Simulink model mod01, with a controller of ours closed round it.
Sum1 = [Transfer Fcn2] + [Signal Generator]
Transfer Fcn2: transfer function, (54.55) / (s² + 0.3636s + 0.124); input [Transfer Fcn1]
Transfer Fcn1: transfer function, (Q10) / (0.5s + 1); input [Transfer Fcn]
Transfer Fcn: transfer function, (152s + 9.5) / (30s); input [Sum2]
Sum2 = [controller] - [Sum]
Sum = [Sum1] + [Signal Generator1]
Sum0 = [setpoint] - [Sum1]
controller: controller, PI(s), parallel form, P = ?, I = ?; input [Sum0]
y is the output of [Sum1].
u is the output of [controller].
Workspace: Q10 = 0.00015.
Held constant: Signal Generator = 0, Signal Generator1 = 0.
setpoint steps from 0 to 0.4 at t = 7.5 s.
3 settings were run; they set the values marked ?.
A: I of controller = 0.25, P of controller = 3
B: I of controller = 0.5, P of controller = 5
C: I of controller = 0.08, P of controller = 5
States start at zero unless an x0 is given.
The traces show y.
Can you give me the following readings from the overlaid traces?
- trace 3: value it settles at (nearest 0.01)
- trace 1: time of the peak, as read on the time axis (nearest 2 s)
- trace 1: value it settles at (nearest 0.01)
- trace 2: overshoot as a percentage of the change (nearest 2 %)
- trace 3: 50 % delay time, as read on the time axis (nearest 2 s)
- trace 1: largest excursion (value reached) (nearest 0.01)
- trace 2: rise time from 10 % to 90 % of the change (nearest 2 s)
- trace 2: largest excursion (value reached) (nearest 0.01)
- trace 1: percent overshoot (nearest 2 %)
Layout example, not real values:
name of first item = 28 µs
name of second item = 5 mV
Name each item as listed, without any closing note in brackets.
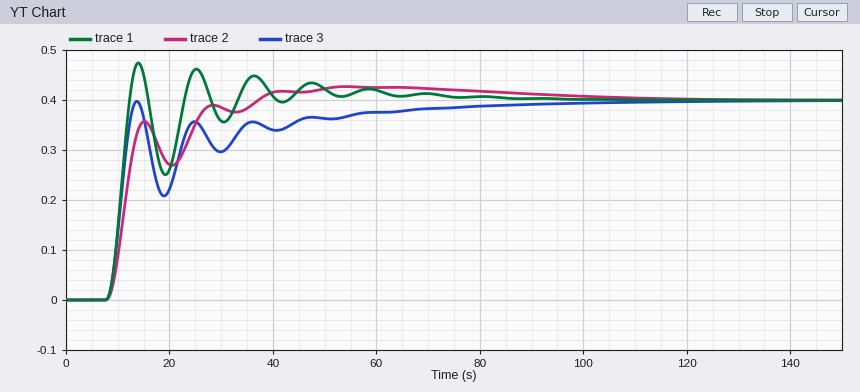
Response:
trace 3: value it settles at = 0.40
trace 1: time of the peak, as read on the time axis = 14 s
trace 1: value it settles at = 0.40
trace 2: overshoot as a percentage of the change = 6 %
trace 3: 50 % delay time, as read on the time axis = 10 s
trace 1: largest excursion (value reached) = 0.47
trace 2: rise time from 10 % to 90 % of the change = 16 s
trace 2: largest excursion (value reached) = 0.43
trace 1: percent overshoot = 18 %
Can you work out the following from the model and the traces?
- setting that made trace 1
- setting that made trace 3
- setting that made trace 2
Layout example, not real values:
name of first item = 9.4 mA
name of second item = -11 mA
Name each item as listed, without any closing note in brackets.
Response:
setting that made trace 1 = B
setting that made trace 3 = C
setting that made trace 2 = A
